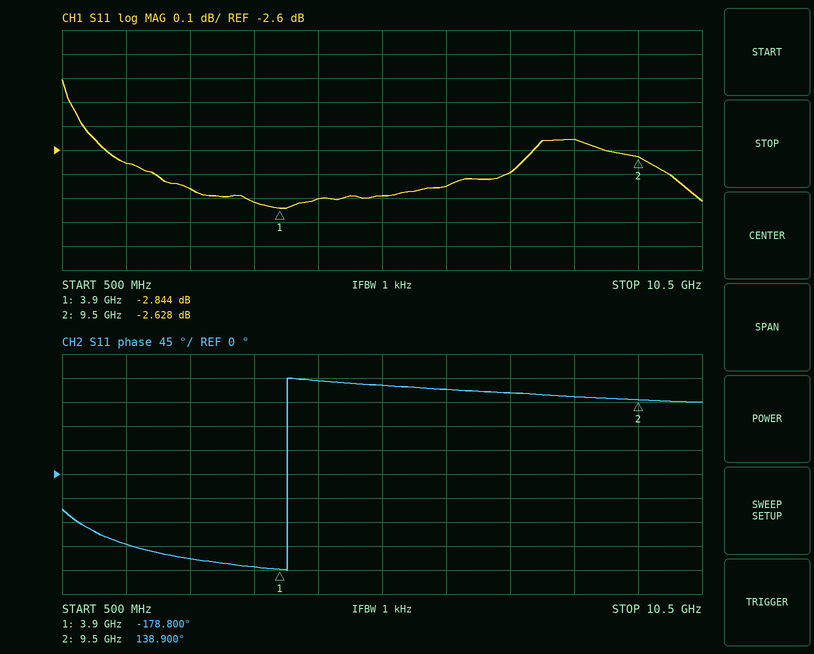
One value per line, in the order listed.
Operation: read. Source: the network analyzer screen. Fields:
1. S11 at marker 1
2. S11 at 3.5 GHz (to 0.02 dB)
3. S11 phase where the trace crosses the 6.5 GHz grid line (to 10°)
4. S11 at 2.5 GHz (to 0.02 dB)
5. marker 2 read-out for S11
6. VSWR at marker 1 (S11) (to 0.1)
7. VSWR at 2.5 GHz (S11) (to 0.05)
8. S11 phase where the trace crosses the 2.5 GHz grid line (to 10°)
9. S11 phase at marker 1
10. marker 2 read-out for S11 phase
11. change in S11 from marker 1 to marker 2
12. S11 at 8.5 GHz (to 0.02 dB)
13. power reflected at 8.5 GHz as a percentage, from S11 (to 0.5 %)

-2.844 dB
-2.82 dB
160°
-2.76 dB
-2.628 dB
6.2
6.35
-160°
-178.800°
138.900°
0.216 dB
-2.56 dB
55.5 %
